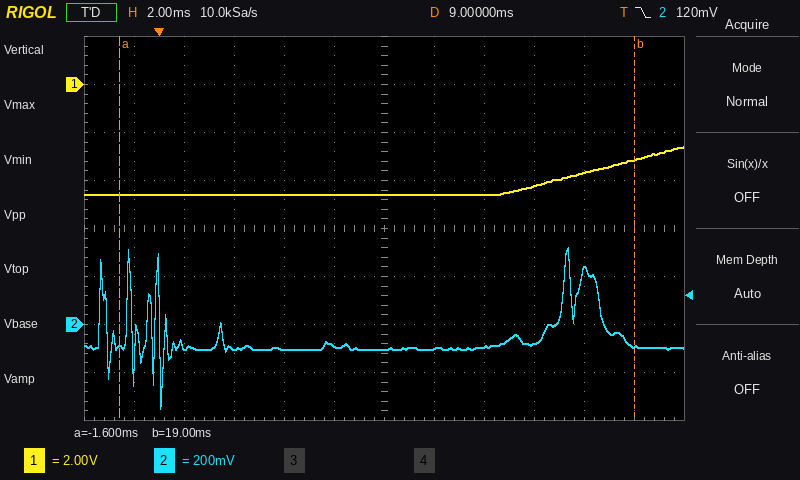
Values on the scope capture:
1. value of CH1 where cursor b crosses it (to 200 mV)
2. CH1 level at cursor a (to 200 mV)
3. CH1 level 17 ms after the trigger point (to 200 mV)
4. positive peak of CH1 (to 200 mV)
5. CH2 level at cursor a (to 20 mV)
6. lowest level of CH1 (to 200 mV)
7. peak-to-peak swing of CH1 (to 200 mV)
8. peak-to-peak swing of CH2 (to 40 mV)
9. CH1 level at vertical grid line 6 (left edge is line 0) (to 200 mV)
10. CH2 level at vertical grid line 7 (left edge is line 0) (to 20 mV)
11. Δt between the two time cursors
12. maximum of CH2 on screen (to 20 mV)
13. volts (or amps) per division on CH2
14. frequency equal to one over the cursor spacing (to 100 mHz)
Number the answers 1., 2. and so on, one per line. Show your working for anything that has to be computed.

1. -3.2 V
2. -4.6 V
3. -3.6 V
4. -2.6 V
5. -100 mV
6. -4.6 V
7. -2.6 V − (-4.6 V) = 2.0 V
8. 680 mV
9. -4.6 V
10. -100 mV
11. 19 ms − (-1.6 ms) = 20.6 ms
12. 320 mV
13. 200 mV
14. 1 / 20.6 ms ≈ 48.5 Hz
